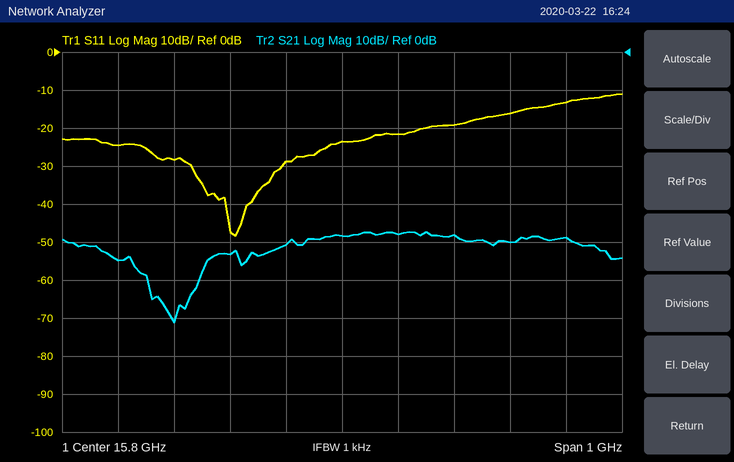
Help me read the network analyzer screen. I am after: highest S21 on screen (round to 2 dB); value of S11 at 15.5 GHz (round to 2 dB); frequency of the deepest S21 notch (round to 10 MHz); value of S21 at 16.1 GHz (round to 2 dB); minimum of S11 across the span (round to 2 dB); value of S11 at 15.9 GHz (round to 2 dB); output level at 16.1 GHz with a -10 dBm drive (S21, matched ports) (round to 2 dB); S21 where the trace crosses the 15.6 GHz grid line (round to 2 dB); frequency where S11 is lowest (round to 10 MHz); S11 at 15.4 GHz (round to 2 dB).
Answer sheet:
-48 dB
-28 dB
15.50 GHz
-50 dB
-48 dB
-22 dB
-60 dBm
-54 dB
15.61 GHz
-24 dB
